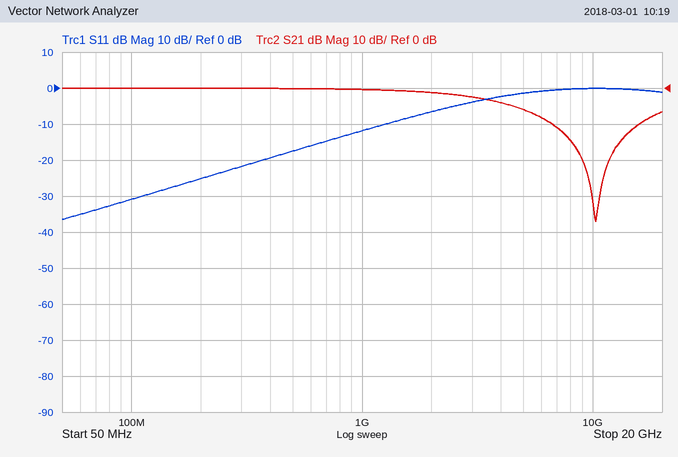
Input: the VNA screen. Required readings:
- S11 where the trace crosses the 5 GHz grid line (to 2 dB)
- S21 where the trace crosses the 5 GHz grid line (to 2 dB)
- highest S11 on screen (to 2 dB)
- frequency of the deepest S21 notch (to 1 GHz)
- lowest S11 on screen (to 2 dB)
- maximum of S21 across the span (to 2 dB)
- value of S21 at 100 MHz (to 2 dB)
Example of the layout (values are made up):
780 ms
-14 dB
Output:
-2 dB
-6 dB
0 dB
10 GHz
-36 dB
0 dB
0 dB
